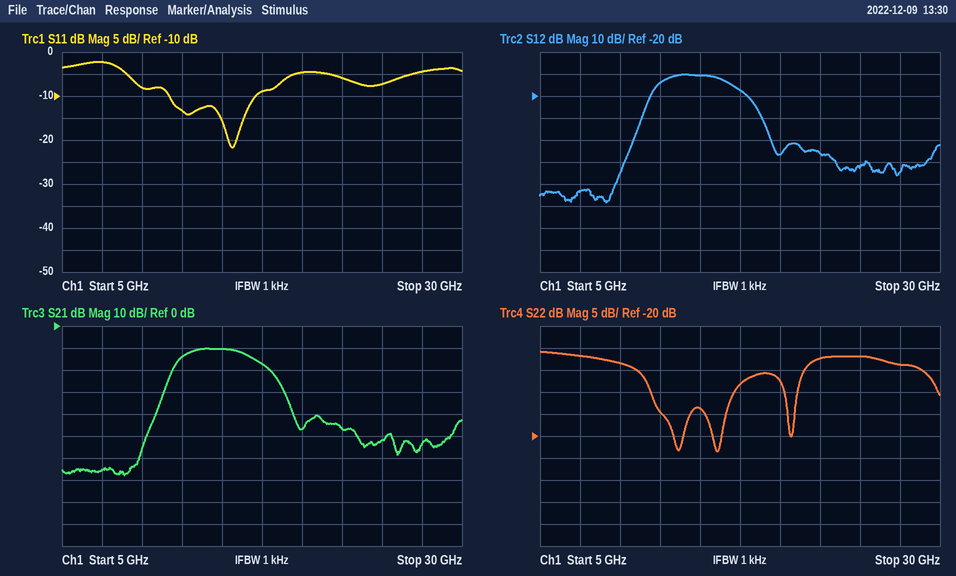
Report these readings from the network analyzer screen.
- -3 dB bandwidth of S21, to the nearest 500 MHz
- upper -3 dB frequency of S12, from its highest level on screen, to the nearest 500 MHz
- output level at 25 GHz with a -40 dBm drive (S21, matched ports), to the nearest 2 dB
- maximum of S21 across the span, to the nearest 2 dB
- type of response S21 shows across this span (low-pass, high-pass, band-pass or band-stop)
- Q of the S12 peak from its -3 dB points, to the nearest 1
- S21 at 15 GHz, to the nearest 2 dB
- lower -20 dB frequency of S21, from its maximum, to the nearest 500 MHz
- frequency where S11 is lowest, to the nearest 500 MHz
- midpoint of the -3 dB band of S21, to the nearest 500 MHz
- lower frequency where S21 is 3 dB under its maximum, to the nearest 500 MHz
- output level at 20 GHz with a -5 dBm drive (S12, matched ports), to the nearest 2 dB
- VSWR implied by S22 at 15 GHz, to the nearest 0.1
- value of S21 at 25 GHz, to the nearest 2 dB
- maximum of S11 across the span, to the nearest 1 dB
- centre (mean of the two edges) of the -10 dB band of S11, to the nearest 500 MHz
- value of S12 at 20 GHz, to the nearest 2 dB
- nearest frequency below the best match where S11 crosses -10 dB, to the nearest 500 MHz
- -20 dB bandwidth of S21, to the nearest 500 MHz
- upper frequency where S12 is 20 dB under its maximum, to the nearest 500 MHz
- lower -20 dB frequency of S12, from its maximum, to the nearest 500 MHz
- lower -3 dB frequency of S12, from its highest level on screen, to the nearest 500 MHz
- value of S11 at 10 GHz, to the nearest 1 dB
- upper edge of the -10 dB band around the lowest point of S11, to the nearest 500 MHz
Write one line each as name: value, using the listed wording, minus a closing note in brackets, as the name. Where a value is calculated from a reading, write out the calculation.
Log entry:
-3 dB bandwidth of S21, to the nearest 500 MHz: 16.5 GHz − 12.5 GHz = 4.0 GHz
upper -3 dB frequency of S12, from its highest level on screen, to the nearest 500 MHz: 16.5 GHz
output level at 25 GHz with a -40 dBm drive (S21, matched ports), to the nearest 2 dB: -40 dBm + (-52 dB) = -92 dBm
maximum of S21 across the span, to the nearest 2 dB: -10 dB
type of response S21 shows across this span: band-pass
Q of the S12 peak from its -3 dB points, to the nearest 1: 14.5 GHz / 4 GHz ≈ 4
S21 at 15 GHz, to the nearest 2 dB: -10 dB
lower -20 dB frequency of S21, from its maximum, to the nearest 500 MHz: 11.5 GHz
frequency where S11 is lowest, to the nearest 500 MHz: 15.5 GHz
midpoint of the -3 dB band of S21, to the nearest 500 MHz: 14.5 GHz
lower frequency where S21 is 3 dB under its maximum, to the nearest 500 MHz: 12.5 GHz
output level at 20 GHz with a -5 dBm drive (S12, matched ports), to the nearest 2 dB: -5 dBm + (-46 dB) = -52 dBm
VSWR implied by S22 at 15 GHz, to the nearest 0.1: |Γ| = 10^(-14/20) = 0.1995; VSWR = (1 + 0.1995)/(1 − 0.1995) ≈ 1.5
value of S21 at 25 GHz, to the nearest 2 dB: -52 dB
maximum of S11 across the span, to the nearest 1 dB: -2 dB
centre (mean of the two edges) of the -10 dB band of S11, to the nearest 500 MHz: 14.5 GHz
value of S12 at 20 GHz, to the nearest 2 dB: -46 dB
nearest frequency below the best match where S11 crosses -10 dB, to the nearest 500 MHz: 11.5 GHz
-20 dB bandwidth of S21, to the nearest 500 MHz: 19.0 GHz − 11.5 GHz = 7.5 GHz
upper frequency where S12 is 20 dB under its maximum, to the nearest 500 MHz: 19.0 GHz
lower -20 dB frequency of S12, from its maximum, to the nearest 500 MHz: 11.5 GHz
lower -3 dB frequency of S12, from its highest level on screen, to the nearest 500 MHz: 12.5 GHz
value of S11 at 10 GHz, to the nearest 1 dB: -8 dB
upper edge of the -10 dB band around the lowest point of S11, to the nearest 500 MHz: 17.0 GHz
